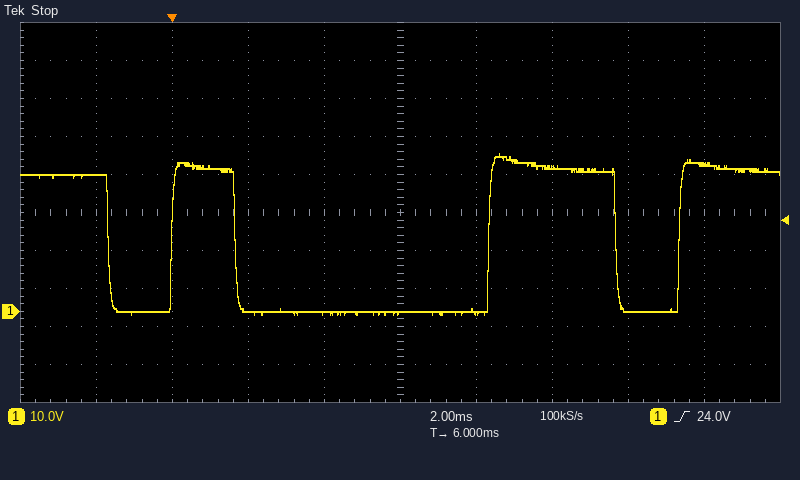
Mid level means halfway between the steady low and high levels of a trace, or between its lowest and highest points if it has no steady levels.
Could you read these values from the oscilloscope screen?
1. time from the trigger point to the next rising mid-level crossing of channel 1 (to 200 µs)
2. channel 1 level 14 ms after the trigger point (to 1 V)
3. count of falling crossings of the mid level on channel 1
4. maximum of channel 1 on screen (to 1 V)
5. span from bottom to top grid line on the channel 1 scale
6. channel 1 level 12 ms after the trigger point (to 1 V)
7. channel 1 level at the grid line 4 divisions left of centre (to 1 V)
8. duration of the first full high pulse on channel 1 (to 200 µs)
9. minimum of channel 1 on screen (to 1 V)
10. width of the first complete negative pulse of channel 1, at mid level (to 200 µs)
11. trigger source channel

8.4 ms
39 V
3
42 V
100 V
0 V
36 V
1.6 ms
-1 V
1.6 ms
channel 1
